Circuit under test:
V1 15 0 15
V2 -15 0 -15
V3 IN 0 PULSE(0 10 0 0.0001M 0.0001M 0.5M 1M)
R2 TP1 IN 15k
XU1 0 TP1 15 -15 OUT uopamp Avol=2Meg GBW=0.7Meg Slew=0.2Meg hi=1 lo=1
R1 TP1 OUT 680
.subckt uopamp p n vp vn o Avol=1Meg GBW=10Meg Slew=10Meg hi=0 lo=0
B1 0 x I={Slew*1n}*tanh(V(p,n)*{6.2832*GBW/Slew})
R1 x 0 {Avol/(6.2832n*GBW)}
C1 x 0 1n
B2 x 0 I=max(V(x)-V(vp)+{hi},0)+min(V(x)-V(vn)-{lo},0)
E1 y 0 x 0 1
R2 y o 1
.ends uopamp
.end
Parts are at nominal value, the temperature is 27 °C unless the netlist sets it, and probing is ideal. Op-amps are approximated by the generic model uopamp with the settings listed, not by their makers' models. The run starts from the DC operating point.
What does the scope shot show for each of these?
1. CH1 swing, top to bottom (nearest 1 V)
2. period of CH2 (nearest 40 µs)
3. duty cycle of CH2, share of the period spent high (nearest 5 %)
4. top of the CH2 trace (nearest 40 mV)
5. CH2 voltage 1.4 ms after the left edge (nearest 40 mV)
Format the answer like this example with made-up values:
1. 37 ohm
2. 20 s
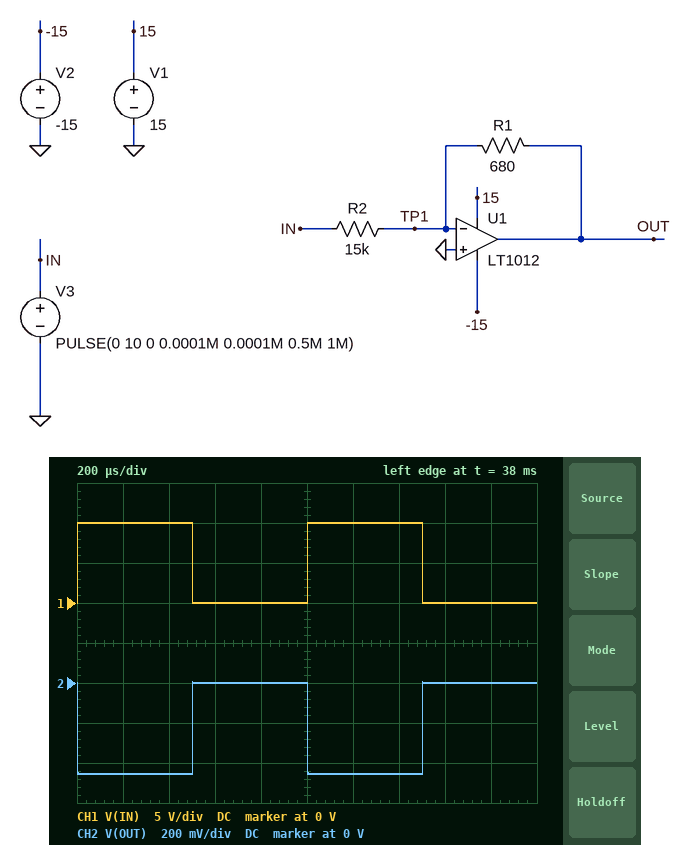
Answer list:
1. 10 V
2. 1.00 ms
3. 50 %
4. 0 V
5. -440 mV
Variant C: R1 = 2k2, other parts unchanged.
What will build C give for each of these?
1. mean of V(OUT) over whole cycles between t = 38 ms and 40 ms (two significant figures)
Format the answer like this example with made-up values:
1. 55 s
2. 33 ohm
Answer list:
1. -730 mV
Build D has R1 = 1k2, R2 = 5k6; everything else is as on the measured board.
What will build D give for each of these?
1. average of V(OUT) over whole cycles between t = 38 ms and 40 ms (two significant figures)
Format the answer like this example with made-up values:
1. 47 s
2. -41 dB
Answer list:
1. -1.1 V
